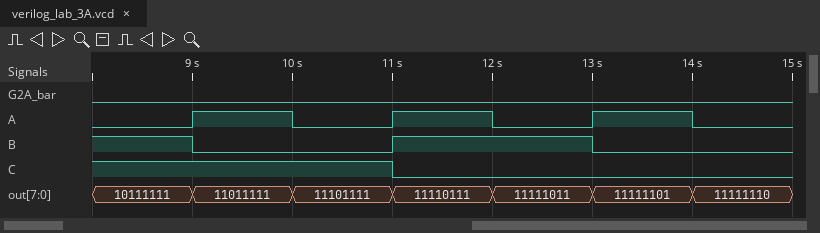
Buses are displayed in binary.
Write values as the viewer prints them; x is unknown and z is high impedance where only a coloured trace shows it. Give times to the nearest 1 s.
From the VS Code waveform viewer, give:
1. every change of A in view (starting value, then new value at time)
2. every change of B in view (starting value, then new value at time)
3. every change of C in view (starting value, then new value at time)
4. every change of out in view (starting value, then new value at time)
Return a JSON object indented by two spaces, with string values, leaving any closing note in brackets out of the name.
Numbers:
{
  "every change of A in view": "0, 1 at 9 s, 0 at 10 s, 1 at 11 s, 0 at 12 s, 1 at 13 s, 0 at 14 s",
  "every change of B in view": "1, 0 at 9 s, 1 at 11 s, 0 at 13 s",
  "every change of C in view": "1, 0 at 11 s",
  "every change of out in view": "10111111, 11011111 at 9 s, 11101111 at 10 s, 11110111 at 11 s, 11111011 at 12 s, 11111101 at 13 s, 11111110 at 14 s"
}
